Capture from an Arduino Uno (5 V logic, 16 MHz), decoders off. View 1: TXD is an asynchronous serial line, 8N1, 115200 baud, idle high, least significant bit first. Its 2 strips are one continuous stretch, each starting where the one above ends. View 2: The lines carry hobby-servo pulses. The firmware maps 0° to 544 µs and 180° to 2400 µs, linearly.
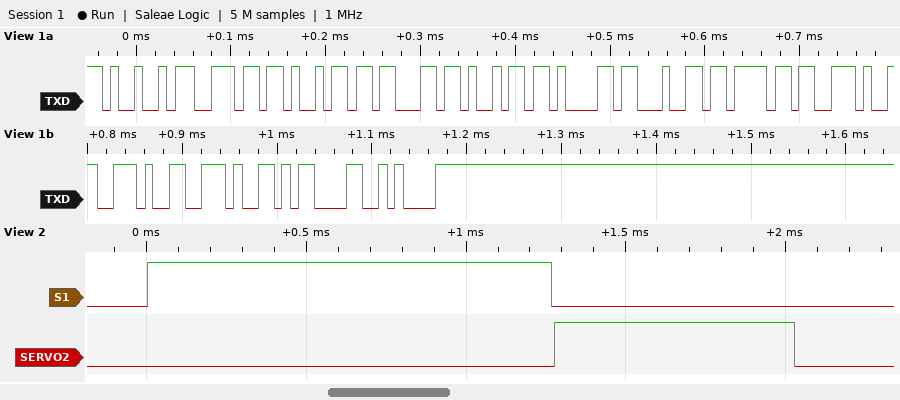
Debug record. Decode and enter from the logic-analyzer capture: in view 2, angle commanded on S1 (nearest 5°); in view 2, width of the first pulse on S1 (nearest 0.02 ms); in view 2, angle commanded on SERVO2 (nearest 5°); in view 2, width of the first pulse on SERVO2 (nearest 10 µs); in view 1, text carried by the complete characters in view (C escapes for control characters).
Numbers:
70°
1.26 ms
20°
750 µs
"Iniciado...\r\n"
